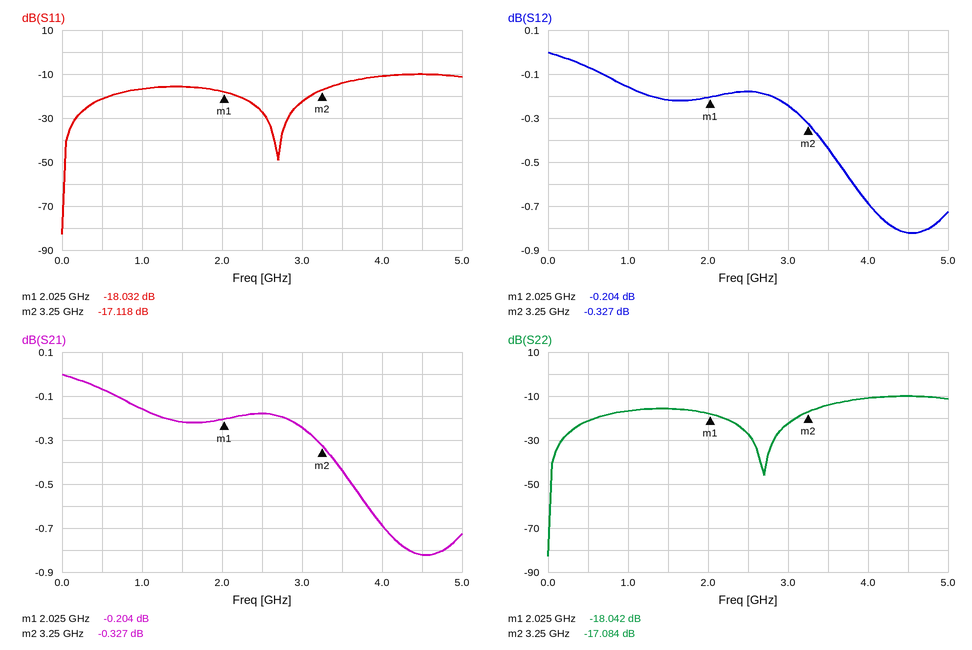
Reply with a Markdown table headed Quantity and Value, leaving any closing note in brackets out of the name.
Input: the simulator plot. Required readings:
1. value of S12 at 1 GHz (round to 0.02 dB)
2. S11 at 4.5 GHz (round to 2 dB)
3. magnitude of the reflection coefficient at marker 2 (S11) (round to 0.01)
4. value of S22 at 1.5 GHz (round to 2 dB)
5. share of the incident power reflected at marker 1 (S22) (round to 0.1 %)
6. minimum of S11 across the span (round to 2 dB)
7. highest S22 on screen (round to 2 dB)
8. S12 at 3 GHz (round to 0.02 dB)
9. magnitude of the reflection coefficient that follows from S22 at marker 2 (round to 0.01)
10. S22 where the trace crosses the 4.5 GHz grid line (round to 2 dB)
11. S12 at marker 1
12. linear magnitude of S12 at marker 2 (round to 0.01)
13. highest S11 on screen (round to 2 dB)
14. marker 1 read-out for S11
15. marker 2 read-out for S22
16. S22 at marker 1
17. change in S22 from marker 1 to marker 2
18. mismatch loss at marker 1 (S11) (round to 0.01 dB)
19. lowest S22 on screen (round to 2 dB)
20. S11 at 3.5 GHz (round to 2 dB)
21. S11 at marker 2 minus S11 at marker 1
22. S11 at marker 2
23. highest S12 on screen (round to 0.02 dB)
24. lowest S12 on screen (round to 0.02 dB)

| Quantity | Value |
|---|---|
| value of S12 at 1 GHz | -0.16 dB |
| S11 at 4.5 GHz | -10 dB |
| magnitude of the reflection coefficient at marker 2 (S11) | 0.14 |
| value of S22 at 1.5 GHz | -16 dB |
| share of the incident power reflected at marker 1 (S22) | 1.6 % |
| minimum of S11 across the span | -82 dB |
| highest S22 on screen | -10 dB |
| S12 at 3 GHz | -0.24 dB |
| magnitude of the reflection coefficient that follows from S22 at marker 2 | 0.14 |
| S22 where the trace crosses the 4.5 GHz grid line | -10 dB |
| S12 at marker 1 | -0.204 dB |
| linear magnitude of S12 at marker 2 | 0.96 |
| highest S11 on screen | -10 dB |
| marker 1 read-out for S11 | -18.032 dB |
| marker 2 read-out for S22 | -17.084 dB |
| S22 at marker 1 | -18.042 dB |
| change in S22 from marker 1 to marker 2 | 0.958 dB |
| mismatch loss at marker 1 (S11) | 0.07 dB |
| lowest S22 on screen | -82 dB |
| S11 at 3.5 GHz | -14 dB |
| S11 at marker 2 minus S11 at marker 1 | 0.914 dB |
| S11 at marker 2 | -17.118 dB |
| highest S12 on screen | 0.00 dB |
| lowest S12 on screen | -0.82 dB |
